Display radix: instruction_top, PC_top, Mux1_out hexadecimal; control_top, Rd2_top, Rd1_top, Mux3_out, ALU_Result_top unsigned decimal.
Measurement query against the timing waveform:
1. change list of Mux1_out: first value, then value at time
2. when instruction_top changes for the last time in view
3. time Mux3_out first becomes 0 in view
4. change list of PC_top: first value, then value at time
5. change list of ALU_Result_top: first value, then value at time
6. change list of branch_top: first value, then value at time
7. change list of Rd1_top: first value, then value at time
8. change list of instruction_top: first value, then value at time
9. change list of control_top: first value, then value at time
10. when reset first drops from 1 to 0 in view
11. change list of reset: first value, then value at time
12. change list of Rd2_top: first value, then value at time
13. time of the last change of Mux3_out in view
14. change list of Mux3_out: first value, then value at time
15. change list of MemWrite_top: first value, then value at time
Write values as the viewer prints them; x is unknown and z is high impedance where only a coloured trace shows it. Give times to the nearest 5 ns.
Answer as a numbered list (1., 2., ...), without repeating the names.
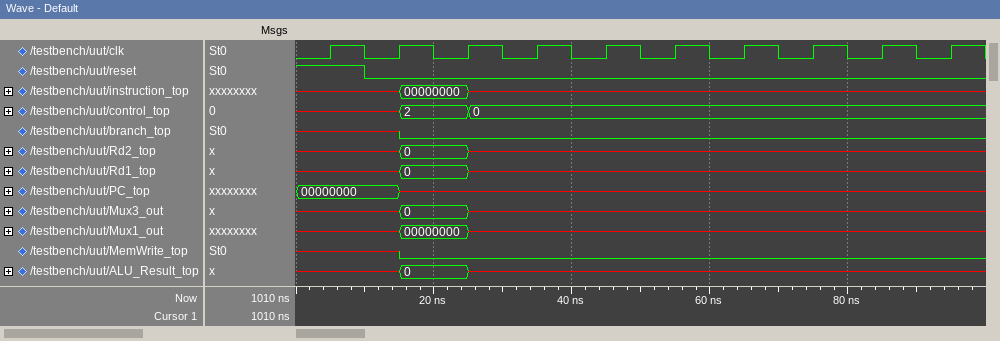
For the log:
1. x, 00000000 at 15 ns, x at 25 ns
2. 25 ns
3. 15 ns
4. 00000000, x at 15 ns
5. x, 0 at 15 ns, x at 25 ns
6. x, 0 at 15 ns
7. x, 0 at 15 ns, x at 25 ns
8. x, 00000000 at 15 ns, x at 25 ns
9. x, 2 at 15 ns, 0 at 25 ns
10. 10 ns
11. 1, 0 at 10 ns
12. x, 0 at 15 ns, x at 25 ns
13. 25 ns
14. x, 0 at 15 ns, x at 25 ns
15. x, 0 at 15 ns
